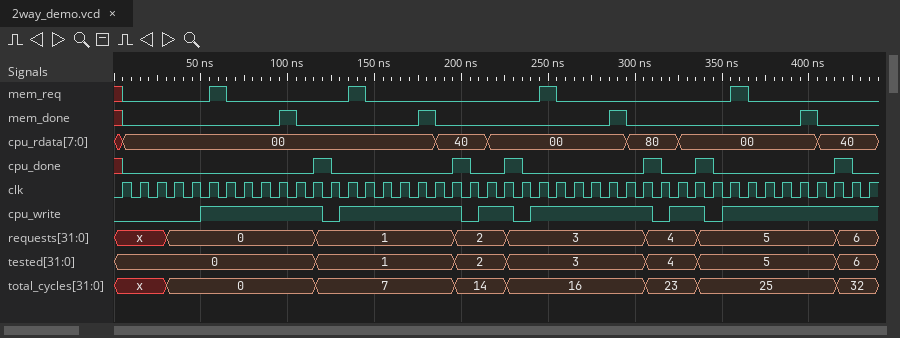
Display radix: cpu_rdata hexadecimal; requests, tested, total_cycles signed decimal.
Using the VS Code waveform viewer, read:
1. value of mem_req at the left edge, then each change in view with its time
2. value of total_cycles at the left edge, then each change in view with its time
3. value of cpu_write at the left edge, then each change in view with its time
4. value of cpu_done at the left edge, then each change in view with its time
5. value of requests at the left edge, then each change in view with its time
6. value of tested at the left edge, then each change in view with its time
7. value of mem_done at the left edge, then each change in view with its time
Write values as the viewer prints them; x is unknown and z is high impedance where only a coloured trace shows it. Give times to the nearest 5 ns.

x, 0 at 5 ns, 1 at 55 ns, 0 at 65 ns, 1 at 135 ns, 0 at 145 ns, 1 at 245 ns, 0 at 255 ns, 1 at 355 ns, 0 at 365 ns
x, 0 at 30 ns, 7 at 115 ns, 14 at 195 ns, 16 at 225 ns, 23 at 305 ns, 25 at 335 ns, 32 at 415 ns
0, 1 at 50 ns, 0 at 120 ns, 1 at 130 ns, 0 at 200 ns, 1 at 210 ns, 0 at 230 ns, 1 at 240 ns, 0 at 310 ns, 1 at 320 ns, 0 at 340 ns, 1 at 350 ns
x, 0 at 5 ns, 1 at 115 ns, 0 at 125 ns, 1 at 195 ns, 0 at 205 ns, 1 at 225 ns, 0 at 235 ns, 1 at 305 ns, 0 at 315 ns, 1 at 335 ns, 0 at 345 ns, 1 at 415 ns, 0 at 425 ns
x, 0 at 30 ns, 1 at 115 ns, 2 at 195 ns, 3 at 225 ns, 4 at 305 ns, 5 at 335 ns, 6 at 415 ns
0, 1 at 115 ns, 2 at 195 ns, 3 at 225 ns, 4 at 305 ns, 5 at 335 ns, 6 at 415 ns
x, 0 at 5 ns, 1 at 95 ns, 0 at 105 ns, 1 at 175 ns, 0 at 185 ns, 1 at 285 ns, 0 at 295 ns, 1 at 395 ns, 0 at 405 ns
